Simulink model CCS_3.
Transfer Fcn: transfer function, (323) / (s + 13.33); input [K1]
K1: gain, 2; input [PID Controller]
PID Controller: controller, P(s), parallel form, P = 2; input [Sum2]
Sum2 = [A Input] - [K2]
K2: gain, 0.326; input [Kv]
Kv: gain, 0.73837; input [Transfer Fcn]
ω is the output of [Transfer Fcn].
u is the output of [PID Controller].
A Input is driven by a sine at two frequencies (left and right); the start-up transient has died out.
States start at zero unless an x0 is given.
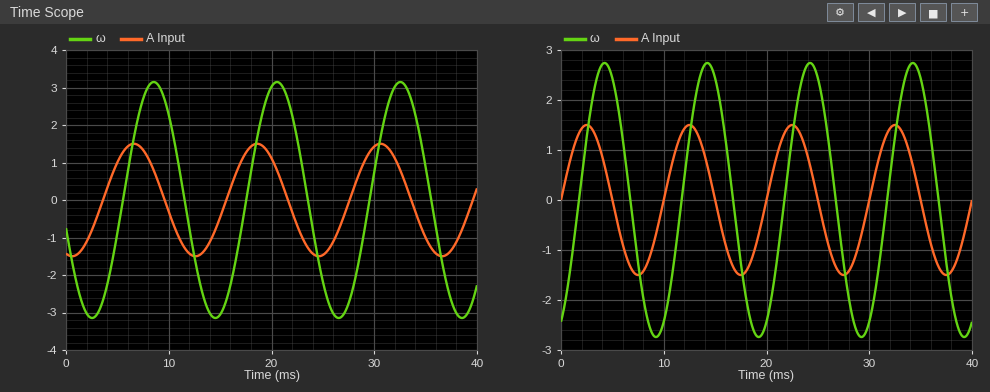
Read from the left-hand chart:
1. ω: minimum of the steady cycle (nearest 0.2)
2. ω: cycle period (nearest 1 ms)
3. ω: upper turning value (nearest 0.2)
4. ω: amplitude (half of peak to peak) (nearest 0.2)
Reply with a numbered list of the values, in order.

1. -3.2
2. 12 ms
3. 3.2
4. 3.2
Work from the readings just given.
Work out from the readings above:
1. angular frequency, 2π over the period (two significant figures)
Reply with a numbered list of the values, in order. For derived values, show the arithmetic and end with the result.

1. 2π / 12 = 0.52 rad/ms
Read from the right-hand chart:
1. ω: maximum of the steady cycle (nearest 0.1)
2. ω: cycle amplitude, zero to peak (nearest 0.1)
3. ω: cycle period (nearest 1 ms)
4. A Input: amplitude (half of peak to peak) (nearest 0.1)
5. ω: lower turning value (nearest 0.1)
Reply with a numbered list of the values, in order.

1. 2.7
2. 2.7
3. 10 ms
4. 1.5
5. -2.7
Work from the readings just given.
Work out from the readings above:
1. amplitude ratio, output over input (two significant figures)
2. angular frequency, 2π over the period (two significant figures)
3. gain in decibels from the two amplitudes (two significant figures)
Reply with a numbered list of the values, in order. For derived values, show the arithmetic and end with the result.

1. 2.7 / 1.5 = 1.8
2. 2π / 10 = 0.63 rad/ms
3. 20 log10(2.7 / 1.5) = 5.1 dB
